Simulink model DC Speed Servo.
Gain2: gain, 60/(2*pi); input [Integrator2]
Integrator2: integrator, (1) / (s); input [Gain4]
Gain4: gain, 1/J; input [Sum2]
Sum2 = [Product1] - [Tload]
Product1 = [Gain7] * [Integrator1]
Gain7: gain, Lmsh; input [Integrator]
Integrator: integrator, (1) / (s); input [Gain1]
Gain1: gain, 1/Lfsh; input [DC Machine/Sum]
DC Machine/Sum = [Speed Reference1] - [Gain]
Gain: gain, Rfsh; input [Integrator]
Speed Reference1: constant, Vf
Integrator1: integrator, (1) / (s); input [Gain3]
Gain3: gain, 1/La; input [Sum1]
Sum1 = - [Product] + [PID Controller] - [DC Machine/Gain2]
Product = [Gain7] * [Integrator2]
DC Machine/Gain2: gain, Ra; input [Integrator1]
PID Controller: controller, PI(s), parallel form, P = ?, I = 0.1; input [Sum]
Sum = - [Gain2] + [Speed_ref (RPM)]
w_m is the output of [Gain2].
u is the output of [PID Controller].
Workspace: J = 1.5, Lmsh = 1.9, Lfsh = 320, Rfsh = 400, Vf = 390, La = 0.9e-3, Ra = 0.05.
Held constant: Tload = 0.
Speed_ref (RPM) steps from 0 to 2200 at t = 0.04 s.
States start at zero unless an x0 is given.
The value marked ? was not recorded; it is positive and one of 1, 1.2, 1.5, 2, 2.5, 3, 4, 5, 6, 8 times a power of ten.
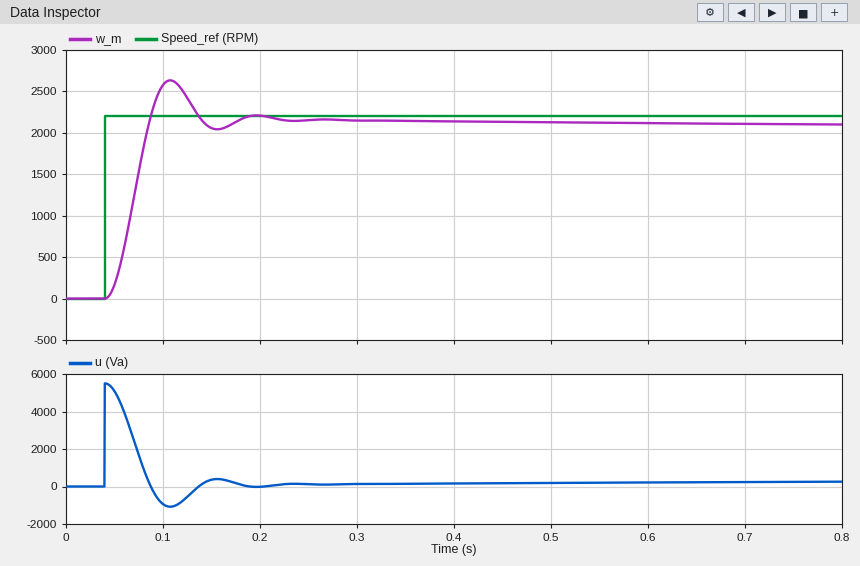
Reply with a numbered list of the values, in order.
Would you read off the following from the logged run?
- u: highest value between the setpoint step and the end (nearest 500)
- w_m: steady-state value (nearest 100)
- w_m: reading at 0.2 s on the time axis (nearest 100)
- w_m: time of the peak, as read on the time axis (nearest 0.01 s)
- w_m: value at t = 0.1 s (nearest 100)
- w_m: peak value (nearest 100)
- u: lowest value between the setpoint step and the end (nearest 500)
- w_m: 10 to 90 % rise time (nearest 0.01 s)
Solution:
1. 5500
2. 2100
3. 2200
4. 0.11 s
5. 2600
6. 2600
7. -1000
8. 0.03 s
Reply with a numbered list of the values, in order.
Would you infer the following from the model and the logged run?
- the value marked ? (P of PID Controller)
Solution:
1. 2.5
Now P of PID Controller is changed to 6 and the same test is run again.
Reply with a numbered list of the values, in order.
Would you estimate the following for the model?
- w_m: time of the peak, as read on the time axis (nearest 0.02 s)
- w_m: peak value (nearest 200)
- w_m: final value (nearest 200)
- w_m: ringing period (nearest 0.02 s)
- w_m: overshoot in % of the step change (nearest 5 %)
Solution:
1. 0.08 s
2. 3000
3. 2200
4. 0.06 s
5. 40 %
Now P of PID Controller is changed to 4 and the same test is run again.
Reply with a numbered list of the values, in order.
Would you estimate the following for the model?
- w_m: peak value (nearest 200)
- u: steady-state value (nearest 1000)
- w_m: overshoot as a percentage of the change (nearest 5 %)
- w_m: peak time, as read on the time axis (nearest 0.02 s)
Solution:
1. 2800
2. 0
3. 35 %
4. 0.10 s
